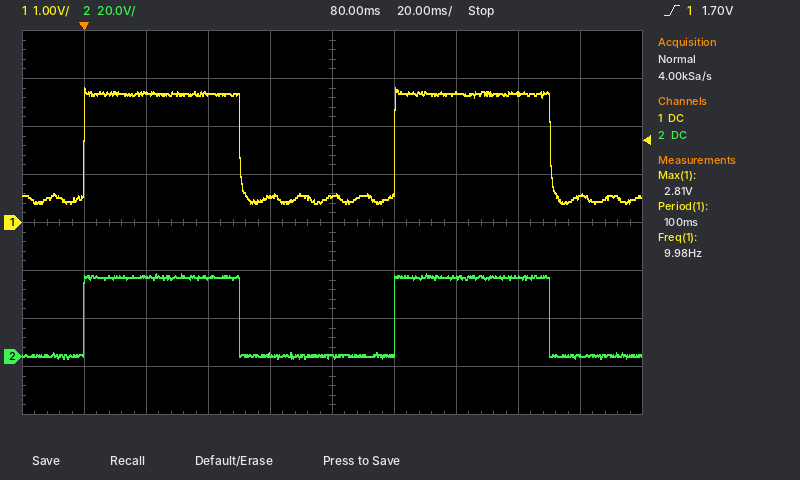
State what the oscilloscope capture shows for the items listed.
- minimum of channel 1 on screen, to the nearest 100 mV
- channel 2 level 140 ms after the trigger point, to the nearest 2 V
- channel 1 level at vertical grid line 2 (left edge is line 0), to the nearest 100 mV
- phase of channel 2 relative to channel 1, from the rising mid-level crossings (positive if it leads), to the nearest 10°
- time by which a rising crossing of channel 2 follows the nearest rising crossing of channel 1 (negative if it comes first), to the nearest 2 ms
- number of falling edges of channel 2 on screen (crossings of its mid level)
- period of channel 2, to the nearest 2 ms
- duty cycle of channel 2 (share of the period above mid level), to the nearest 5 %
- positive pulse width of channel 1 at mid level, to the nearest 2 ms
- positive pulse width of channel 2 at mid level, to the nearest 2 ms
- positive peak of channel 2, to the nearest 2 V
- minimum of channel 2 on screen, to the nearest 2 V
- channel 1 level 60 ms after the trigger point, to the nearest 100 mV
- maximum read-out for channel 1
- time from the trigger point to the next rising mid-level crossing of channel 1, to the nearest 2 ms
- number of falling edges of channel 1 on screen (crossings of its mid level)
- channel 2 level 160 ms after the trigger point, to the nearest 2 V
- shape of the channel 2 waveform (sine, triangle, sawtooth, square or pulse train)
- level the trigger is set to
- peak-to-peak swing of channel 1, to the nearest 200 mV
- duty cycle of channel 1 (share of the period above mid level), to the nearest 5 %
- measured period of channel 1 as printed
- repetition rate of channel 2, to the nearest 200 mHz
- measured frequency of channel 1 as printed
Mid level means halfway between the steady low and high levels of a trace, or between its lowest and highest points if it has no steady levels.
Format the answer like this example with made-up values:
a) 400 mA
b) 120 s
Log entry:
a) 400 mV
b) 34 V
c) 2.7 V
d) 0°
e) 0 ms
f) 2
g) 100 ms
h) 50 %
i) 50 ms
j) 50 ms
k) 34 V
l) 0 V
m) 500 mV
n) 2.81 V
o) 100 ms
p) 2
q) 0 V
r) square
s) 1.70 V
t) 2.4 V
u) 50 %
v) 100 ms
w) 10.0 Hz
x) 9.98 Hz
